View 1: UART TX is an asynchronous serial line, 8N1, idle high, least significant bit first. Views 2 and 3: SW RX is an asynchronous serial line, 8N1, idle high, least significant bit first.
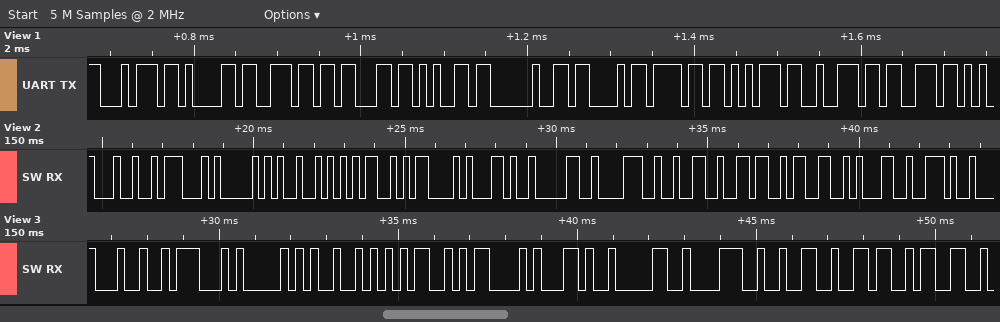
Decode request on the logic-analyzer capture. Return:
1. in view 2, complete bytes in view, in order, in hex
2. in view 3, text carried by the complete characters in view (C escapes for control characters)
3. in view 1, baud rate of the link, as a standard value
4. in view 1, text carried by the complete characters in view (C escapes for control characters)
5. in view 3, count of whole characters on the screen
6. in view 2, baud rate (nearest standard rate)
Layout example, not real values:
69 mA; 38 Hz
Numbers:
0x24 0x47 0x50 0x52 0x4D 0x43 0x2C 0x30 0x38 0x32 0x36 0x33 0x31 0x2E; "$GPRMC,08263"; 115200 baud; "tance Cours"; 12; 4800 baud
